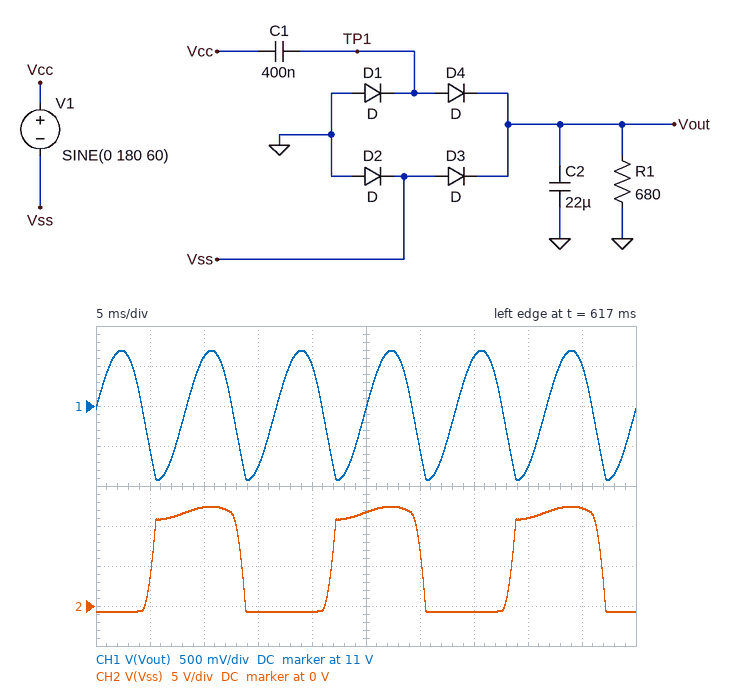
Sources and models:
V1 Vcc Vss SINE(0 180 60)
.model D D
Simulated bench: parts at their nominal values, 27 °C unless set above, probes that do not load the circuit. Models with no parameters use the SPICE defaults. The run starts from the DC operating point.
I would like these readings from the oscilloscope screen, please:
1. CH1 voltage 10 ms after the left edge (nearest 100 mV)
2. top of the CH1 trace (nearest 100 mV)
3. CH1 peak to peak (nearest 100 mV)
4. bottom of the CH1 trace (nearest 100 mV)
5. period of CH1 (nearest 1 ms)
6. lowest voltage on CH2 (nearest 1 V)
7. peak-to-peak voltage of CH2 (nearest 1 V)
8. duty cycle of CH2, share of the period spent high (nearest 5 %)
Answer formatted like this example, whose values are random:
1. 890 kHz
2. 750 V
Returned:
1. 11.6 V
2. 11.7 V
3. 1.6 V
4. 10.1 V
5. 8 ms
6. -1 V
7. 13 V
8. 50 %
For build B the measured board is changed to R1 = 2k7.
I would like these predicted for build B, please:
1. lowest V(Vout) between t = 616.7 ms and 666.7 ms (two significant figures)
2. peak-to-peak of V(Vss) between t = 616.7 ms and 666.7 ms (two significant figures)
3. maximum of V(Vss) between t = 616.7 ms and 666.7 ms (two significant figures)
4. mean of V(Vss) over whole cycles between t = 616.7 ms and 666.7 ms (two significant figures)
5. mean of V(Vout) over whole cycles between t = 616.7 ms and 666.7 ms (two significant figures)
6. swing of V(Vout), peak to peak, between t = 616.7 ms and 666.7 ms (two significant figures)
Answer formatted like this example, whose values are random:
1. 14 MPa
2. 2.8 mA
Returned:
1. 36 V
2. 39 V
3. 38 V
4. 18 V
5. 37 V
6. 2.0 V
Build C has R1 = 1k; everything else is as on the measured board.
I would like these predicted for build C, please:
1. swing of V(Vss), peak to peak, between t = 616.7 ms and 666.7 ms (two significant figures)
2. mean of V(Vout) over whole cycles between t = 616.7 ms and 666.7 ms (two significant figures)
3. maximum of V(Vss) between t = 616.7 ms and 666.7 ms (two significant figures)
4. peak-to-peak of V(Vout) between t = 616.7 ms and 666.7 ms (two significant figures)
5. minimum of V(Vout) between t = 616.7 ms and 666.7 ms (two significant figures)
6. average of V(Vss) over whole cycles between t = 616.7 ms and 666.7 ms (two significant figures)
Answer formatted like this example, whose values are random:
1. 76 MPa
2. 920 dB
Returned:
1. 18 V
2. 16 V
3. 17 V
4. 1.7 V
5. 15 V
6. 7.8 V
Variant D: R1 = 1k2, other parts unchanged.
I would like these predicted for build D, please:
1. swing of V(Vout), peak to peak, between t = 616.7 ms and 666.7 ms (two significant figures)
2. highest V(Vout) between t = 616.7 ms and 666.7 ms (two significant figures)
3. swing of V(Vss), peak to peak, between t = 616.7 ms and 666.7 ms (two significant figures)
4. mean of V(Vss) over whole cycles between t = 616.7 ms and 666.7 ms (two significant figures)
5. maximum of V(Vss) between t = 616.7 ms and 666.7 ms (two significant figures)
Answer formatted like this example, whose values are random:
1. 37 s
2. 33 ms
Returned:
1. 1.8 V
2. 19 V
3. 21 V
4. 9.2 V
5. 20 V
